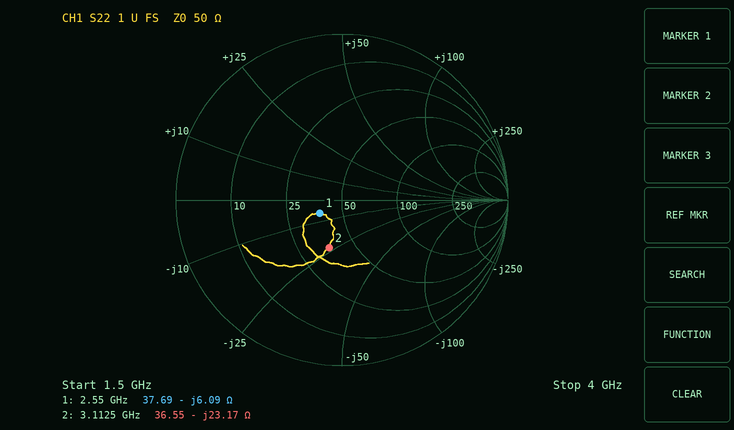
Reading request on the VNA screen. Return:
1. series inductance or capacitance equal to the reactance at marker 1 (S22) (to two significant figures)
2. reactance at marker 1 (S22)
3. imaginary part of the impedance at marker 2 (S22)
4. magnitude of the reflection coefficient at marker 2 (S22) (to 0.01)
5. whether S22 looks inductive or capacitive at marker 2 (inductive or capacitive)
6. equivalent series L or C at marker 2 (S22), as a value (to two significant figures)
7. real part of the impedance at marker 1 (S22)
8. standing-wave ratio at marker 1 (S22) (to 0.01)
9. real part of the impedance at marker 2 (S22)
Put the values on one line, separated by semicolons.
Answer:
10 pF; -6.09 Ω; -23.17 Ω; 0.30; capacitive; 2.2 pF; 37.69 Ω; 1.37; 36.55 Ω
